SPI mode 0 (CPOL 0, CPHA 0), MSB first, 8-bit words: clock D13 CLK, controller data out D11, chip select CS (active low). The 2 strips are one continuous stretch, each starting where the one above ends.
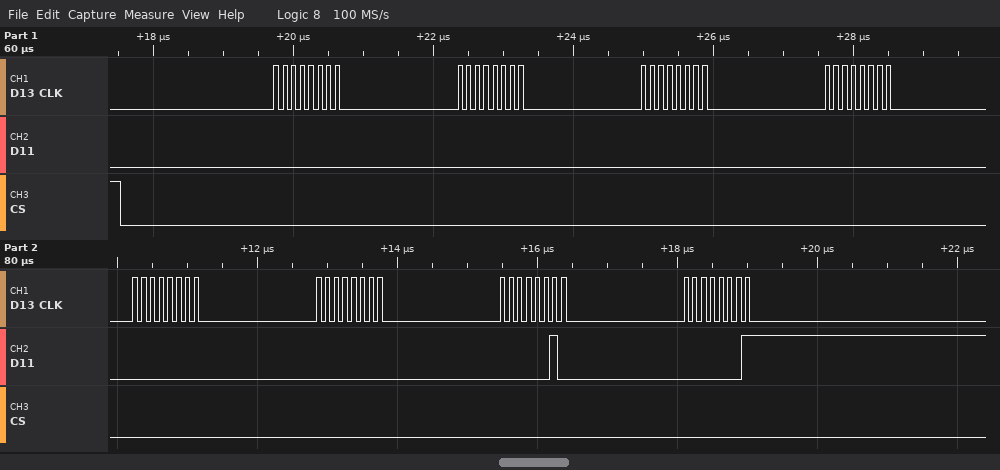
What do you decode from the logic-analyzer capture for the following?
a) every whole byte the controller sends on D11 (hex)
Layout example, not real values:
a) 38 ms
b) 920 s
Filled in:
a) 00 00 00 00 00 00 02 01
